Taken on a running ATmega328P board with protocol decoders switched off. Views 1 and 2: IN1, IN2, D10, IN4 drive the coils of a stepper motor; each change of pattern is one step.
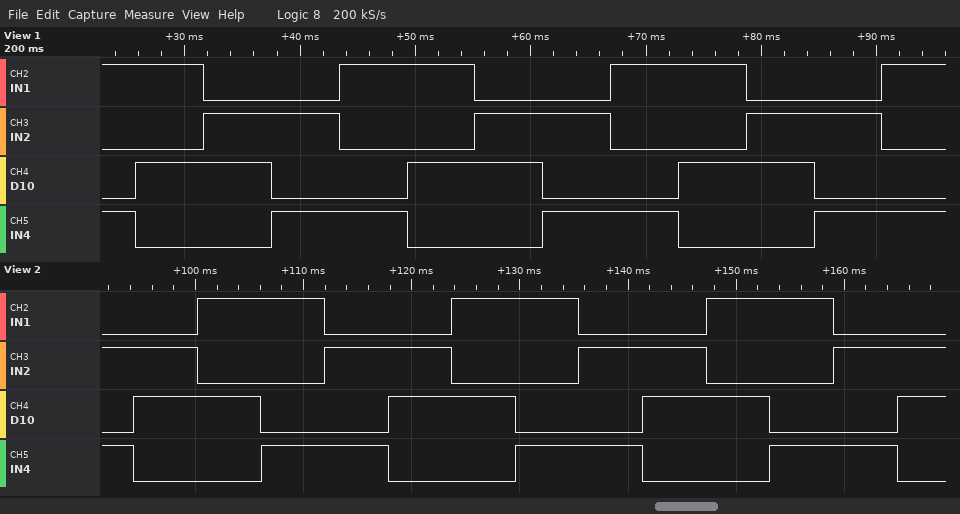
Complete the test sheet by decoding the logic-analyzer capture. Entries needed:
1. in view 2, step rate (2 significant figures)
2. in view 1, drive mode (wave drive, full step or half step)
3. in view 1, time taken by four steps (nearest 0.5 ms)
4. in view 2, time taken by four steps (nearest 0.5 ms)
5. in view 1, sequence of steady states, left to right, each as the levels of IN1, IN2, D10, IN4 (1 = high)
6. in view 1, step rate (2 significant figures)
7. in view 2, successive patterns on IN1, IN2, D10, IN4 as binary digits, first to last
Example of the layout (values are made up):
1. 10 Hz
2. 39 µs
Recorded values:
1. 170 steps/s
2. full step
3. 23.5 ms
4. 23.5 ms
5. 1001 1010 0110 0101 1001 1010 0110 0101 1001 1010 0110 0101 1001
6. 170 steps/s
7. 0101 0110 1010 1001 0101 0110 1010 1001 0101 0110 1010 1001 0101 0110
